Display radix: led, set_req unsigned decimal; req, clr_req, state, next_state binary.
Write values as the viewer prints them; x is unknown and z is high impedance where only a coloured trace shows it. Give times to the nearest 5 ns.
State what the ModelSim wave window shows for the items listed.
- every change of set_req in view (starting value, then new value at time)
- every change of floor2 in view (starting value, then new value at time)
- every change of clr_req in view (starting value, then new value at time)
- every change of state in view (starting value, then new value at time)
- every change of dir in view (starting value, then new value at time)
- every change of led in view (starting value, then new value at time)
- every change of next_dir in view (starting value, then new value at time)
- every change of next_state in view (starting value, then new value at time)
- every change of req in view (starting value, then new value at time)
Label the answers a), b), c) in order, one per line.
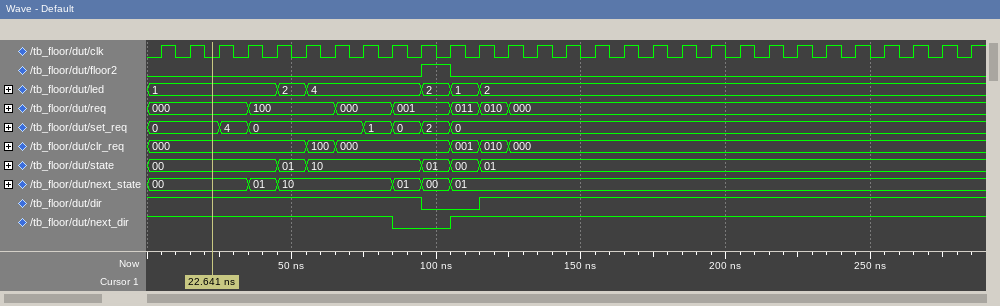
a) 0, 4 at 25 ns, 0 at 35 ns, 1 at 75 ns, 0 at 85 ns, 2 at 95 ns, 0 at 105 ns
b) 0, 1 at 95 ns, 0 at 105 ns
c) 000, 100 at 55 ns, 000 at 65 ns, 001 at 105 ns, 010 at 115 ns, 000 at 125 ns
d) 00, 01 at 45 ns, 10 at 55 ns, 01 at 95 ns, 00 at 105 ns, 01 at 115 ns
e) 1, 0 at 95 ns, 1 at 115 ns
f) 1, 2 at 45 ns, 4 at 55 ns, 2 at 95 ns, 1 at 105 ns, 2 at 115 ns
g) 1, 0 at 85 ns, 1 at 105 ns
h) 00, 01 at 35 ns, 10 at 45 ns, 01 at 85 ns, 00 at 95 ns, 01 at 105 ns
i) 000, 100 at 35 ns, 000 at 65 ns, 001 at 85 ns, 011 at 105 ns, 010 at 115 ns, 000 at 125 ns
